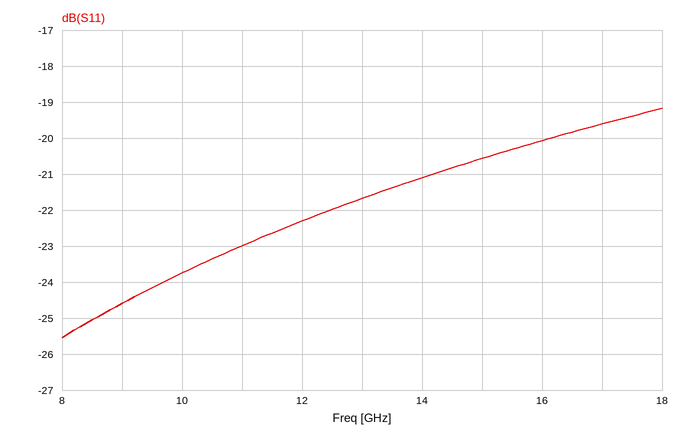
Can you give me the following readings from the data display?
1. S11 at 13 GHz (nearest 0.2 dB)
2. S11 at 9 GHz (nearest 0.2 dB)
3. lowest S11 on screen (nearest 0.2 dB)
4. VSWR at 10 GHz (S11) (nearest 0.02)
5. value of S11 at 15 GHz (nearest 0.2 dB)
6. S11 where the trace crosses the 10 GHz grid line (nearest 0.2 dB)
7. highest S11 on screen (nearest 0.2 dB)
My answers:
-21.6 dB
-24.6 dB
-25.6 dB
1.14
-20.6 dB
-23.8 dB
-19.2 dB
